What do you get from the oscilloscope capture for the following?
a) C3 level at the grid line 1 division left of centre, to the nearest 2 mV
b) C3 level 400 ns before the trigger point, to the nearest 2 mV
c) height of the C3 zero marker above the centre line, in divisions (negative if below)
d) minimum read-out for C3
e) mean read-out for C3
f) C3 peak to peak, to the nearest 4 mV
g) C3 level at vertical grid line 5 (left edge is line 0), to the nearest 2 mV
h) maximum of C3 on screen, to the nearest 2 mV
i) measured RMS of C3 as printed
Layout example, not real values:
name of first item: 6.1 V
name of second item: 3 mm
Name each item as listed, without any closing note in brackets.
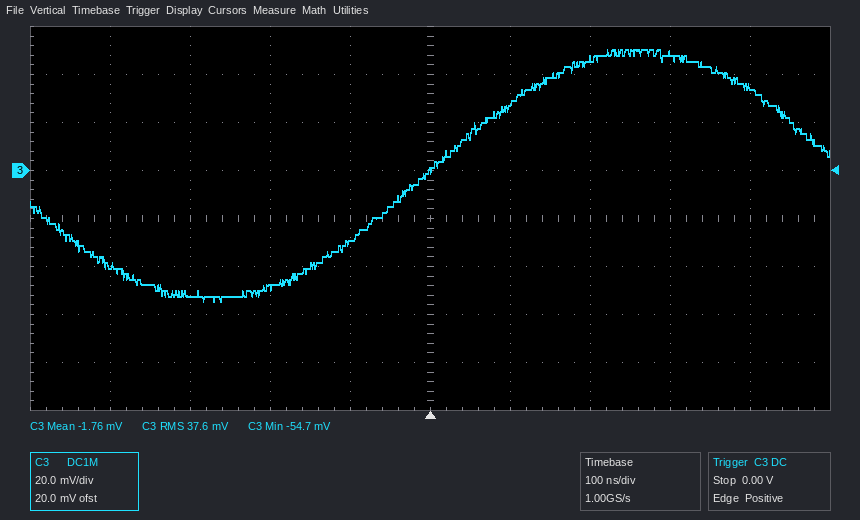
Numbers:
C3 level at the grid line 1 division left of centre, to the nearest 2 mV: -30 mV
C3 level 400 ns before the trigger point, to the nearest 2 mV: -40 mV
height of the C3 zero marker above the centre line, in divisions: +1.0 div
minimum read-out for C3: -54.7 mV
mean read-out for C3: -1.76 mV
C3 peak to peak, to the nearest 4 mV: 104 mV
C3 level at vertical grid line 5 (left edge is line 0), to the nearest 2 mV: 0 mV
maximum of C3 on screen, to the nearest 2 mV: 50 mV
measured RMS of C3 as printed: 37.6 mV
